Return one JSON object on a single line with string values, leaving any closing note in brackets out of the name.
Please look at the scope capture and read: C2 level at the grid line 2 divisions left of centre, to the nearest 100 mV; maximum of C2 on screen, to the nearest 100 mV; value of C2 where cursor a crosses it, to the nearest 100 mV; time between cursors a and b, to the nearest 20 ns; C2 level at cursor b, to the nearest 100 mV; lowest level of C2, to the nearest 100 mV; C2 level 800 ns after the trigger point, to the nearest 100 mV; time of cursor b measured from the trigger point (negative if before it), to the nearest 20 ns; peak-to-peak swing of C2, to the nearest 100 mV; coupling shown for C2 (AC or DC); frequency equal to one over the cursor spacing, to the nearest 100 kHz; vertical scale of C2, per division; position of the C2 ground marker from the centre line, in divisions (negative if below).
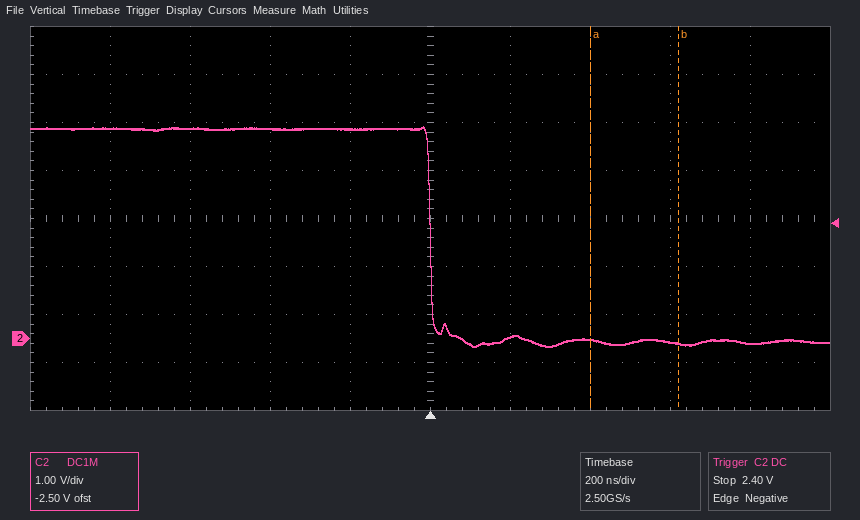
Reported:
{"C2 level at the grid line 2 divisions left of centre, to the nearest 100 mV": "4.4 V", "maximum of C2 on screen, to the nearest 100 mV": "4.4 V", "value of C2 where cursor a crosses it, to the nearest 100 mV": "0.0 V", "time between cursors a and b, to the nearest 20 ns": "220 ns", "C2 level at cursor b, to the nearest 100 mV": "-100 mV", "lowest level of C2, to the nearest 100 mV": "-200 mV", "C2 level 800 ns after the trigger point, to the nearest 100 mV": "-100 mV", "time of cursor b measured from the trigger point (negative if before it), to the nearest 20 ns": "+620 ns", "peak-to-peak swing of C2, to the nearest 100 mV": "4.6 V", "coupling shown for C2": "DC", "frequency equal to one over the cursor spacing, to the nearest 100 kHz": "4.5 MHz", "vertical scale of C2, per division": "1 V", "position of the C2 ground marker from the centre line, in divisions": "-2.5 div"}
